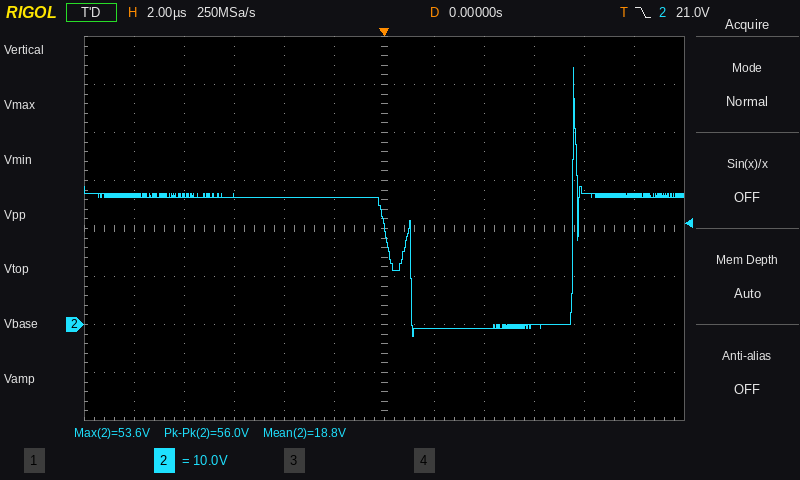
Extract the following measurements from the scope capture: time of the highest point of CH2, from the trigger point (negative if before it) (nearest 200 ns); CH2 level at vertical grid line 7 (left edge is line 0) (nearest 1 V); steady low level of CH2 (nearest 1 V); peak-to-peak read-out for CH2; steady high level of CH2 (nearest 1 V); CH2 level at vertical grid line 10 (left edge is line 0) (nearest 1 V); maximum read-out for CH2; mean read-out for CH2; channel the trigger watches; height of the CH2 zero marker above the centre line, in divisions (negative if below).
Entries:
+7.6 µs
-1 V
-1 V
56.0 V
26 V
28 V
53.6 V
18.8 V
CH2
-2.0 div
